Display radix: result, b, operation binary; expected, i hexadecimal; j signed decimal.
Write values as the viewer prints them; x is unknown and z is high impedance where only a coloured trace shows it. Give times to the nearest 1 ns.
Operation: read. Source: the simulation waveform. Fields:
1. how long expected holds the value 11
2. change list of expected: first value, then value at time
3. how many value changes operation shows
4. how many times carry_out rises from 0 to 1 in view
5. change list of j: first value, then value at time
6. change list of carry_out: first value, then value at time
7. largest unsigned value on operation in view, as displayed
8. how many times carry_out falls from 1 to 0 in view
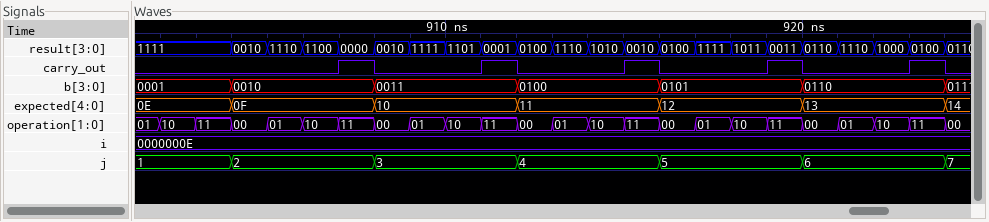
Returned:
4 ns
0E, 0F at 904 ns, 10 at 908 ns, 11 at 912 ns, 12 at 916 ns, 13 at 920 ns, 14 at 924 ns
23
5
1, 2 at 904 ns, 3 at 908 ns, 4 at 912 ns, 5 at 916 ns, 6 at 920 ns, 7 at 924 ns
0, 1 at 907 ns, 0 at 908 ns, 1 at 911 ns, 0 at 912 ns, 1 at 915 ns, 0 at 916 ns, 1 at 919 ns, 0 at 920 ns, 1 at 923 ns, 0 at 924 ns
11
5
